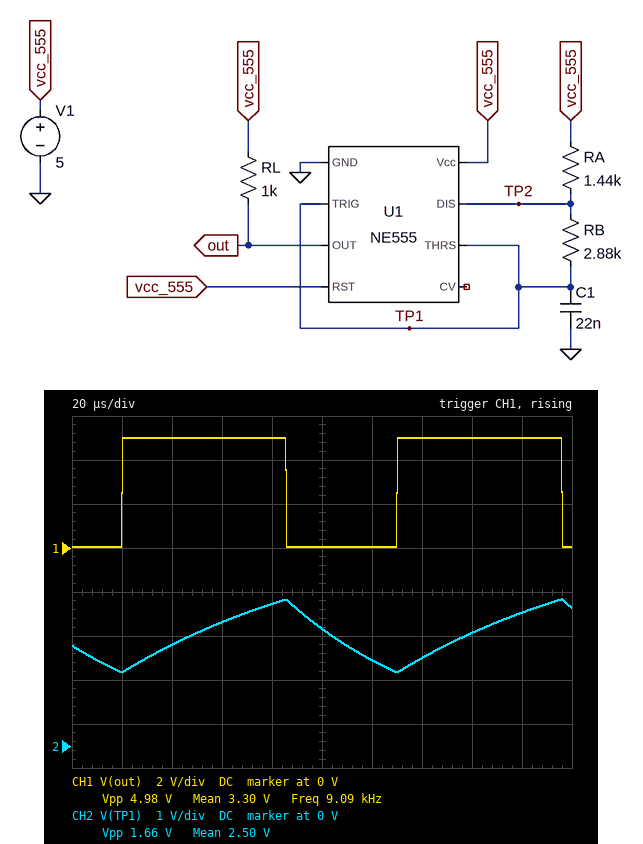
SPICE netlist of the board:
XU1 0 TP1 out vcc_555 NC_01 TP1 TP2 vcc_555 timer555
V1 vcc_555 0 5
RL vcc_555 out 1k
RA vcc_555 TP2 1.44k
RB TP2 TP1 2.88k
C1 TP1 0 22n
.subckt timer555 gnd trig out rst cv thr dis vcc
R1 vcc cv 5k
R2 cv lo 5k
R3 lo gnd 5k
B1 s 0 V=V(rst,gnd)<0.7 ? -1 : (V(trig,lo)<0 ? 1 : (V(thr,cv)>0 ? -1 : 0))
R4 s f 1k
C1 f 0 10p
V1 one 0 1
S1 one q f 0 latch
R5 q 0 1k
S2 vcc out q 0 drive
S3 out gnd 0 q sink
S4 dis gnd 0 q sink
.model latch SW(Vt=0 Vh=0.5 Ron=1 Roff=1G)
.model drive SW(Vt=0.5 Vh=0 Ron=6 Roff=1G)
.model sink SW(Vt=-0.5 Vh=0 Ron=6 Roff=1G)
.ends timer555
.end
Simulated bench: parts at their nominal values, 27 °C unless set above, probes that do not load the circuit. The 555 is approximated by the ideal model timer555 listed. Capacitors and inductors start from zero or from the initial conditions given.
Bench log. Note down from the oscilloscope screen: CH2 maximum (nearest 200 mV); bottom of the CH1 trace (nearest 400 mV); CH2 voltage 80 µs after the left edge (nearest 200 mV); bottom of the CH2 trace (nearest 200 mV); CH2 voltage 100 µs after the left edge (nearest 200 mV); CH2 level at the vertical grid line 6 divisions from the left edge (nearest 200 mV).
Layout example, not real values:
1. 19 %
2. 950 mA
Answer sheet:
1. 3.4 V
2. 0 V
3. 3.2 V
4. 1.6 V
5. 2.6 V
6. 2.0 V
